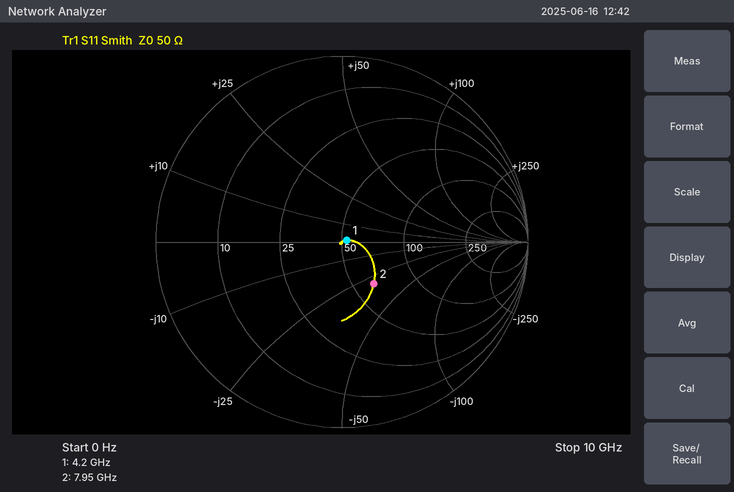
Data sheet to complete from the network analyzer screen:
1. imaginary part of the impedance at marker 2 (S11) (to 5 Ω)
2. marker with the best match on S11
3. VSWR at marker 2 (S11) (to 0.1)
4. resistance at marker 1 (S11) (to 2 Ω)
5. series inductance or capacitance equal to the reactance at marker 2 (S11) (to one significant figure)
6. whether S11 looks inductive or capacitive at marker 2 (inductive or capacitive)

-30 Ω
marker 1
1.8
52 Ω
700 fF
capacitive
